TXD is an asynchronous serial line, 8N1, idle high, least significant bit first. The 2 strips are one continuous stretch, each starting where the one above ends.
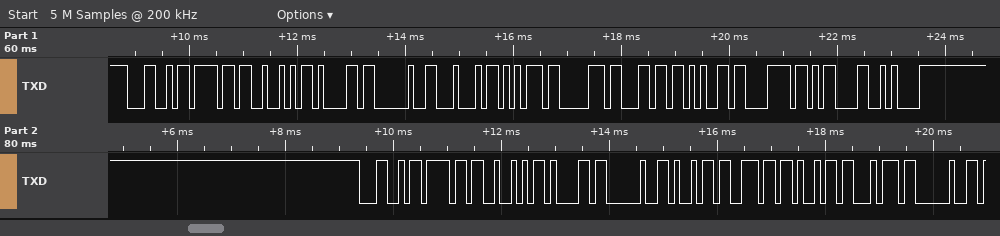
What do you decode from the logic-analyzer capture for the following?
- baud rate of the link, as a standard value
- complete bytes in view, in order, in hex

9600 baud
4C 6F 52 61 20 44 75 70 6C 65 78 0D 0A 4C 6F 52 61 20 69 6E 69 74 20
